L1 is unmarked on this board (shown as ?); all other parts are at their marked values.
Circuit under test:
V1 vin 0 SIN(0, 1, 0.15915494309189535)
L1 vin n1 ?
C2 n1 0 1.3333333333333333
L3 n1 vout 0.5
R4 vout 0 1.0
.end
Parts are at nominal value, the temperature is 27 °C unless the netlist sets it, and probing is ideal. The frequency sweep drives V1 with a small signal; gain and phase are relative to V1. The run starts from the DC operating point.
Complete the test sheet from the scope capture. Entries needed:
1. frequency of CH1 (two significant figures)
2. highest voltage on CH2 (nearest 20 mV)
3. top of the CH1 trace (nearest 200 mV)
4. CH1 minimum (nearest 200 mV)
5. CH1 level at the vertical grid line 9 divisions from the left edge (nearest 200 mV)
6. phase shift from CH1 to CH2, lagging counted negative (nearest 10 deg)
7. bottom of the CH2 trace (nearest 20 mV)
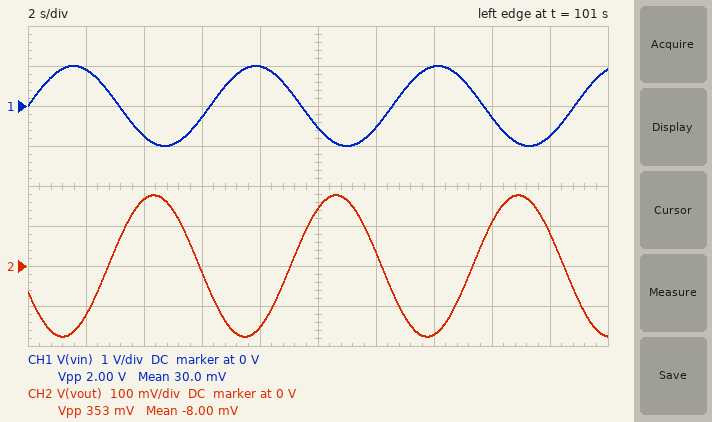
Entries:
160 mHz
180 mV
1.0 V
-1.0 V
-800 mV
-160 deg
-180 mV
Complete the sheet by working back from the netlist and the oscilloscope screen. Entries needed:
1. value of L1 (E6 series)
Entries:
4.7 H
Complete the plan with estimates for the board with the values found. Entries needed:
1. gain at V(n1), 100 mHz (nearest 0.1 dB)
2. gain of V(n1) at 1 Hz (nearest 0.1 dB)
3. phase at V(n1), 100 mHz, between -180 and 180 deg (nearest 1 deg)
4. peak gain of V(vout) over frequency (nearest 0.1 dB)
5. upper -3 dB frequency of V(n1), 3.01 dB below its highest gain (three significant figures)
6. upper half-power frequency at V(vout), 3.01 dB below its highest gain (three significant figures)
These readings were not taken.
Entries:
-8.8 dB
-47.5 dB
-103 deg
0 dB
41.8 mHz
41.1 mHz
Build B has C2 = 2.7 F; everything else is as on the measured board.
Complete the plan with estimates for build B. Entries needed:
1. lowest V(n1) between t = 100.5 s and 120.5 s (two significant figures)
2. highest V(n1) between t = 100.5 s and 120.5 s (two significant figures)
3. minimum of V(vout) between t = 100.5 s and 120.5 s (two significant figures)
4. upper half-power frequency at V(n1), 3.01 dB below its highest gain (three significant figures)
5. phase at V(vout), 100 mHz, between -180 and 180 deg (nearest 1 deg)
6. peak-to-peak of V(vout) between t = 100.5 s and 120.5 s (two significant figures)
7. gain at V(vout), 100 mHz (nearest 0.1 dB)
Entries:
-95 mV
95 mV
-85 mV
49.0 mHz
-157 deg
170 mV
-12.8 dB
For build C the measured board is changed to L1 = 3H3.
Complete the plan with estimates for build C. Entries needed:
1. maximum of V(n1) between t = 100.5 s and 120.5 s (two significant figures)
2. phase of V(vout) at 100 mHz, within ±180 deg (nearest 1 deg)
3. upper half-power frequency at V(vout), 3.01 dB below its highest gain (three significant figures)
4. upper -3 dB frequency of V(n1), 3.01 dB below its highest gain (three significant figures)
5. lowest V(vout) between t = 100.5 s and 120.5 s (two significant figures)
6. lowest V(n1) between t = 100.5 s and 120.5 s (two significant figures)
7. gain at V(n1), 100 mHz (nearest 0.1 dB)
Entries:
300 mV
-112 deg
64.0 mHz
66.4 mHz
-270 mV
-300 mV
-5.5 dB
